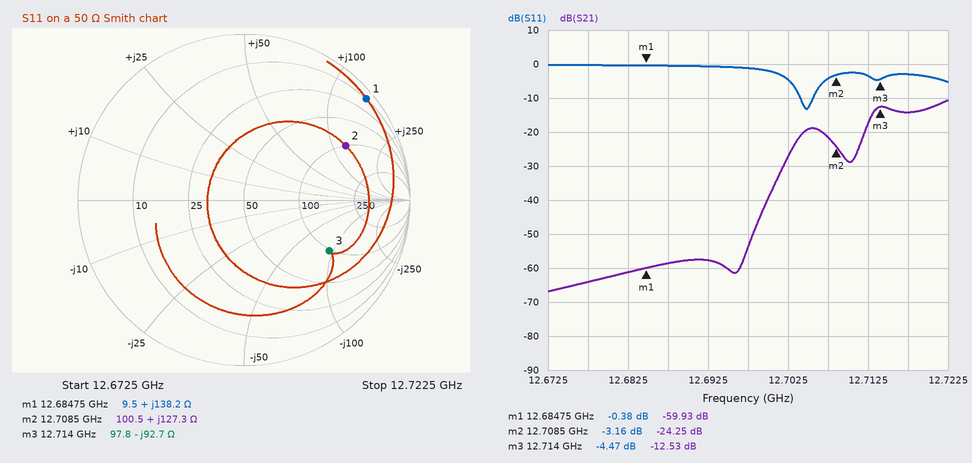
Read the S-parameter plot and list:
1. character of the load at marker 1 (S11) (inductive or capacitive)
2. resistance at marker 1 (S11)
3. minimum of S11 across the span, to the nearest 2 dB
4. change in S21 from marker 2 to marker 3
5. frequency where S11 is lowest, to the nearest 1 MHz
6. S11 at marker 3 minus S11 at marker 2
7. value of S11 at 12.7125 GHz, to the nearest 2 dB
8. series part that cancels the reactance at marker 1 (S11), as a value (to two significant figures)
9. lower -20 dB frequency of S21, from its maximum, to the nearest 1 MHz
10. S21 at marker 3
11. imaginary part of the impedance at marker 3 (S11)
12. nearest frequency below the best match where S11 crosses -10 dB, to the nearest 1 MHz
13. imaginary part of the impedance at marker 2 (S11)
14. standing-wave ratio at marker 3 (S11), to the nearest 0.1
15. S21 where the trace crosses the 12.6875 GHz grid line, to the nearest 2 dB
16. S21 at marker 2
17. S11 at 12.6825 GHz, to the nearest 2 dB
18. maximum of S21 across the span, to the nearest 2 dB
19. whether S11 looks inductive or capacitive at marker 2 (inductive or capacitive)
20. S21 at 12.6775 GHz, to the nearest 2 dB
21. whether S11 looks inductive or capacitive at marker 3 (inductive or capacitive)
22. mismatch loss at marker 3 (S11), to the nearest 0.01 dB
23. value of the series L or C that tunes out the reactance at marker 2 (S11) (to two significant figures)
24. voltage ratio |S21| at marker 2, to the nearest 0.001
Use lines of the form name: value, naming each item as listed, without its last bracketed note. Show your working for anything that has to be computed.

character of the load at marker 1 (S11): inductive
resistance at marker 1: 9.5 Ω
minimum of S11 across the span, to the nearest 2 dB: -14 dB
change in S21 from marker 2 to marker 3: -12.53 − (-24.25) = 11.72 dB
frequency where S11 is lowest, to the nearest 1 MHz: 12.705 GHz
S11 at marker 3 minus S11 at marker 2: -4.47 − (-3.16) = -1.31 dB
value of S11 at 12.7125 GHz, to the nearest 2 dB: -4 dB
series part that cancels the reactance at marker 1 (S11), as a value: C = 1/(2π × 12.68475 GHz × 138.2 Ω) ≈ 91 fF
lower -20 dB frequency of S21, from its maximum, to the nearest 1 MHz: 12.702 GHz
S21 at marker 3: -12.53 dB
imaginary part of the impedance at marker 3: -92.7 Ω
nearest frequency below the best match where S11 crosses -10 dB, to the nearest 1 MHz: 12.704 GHz
imaginary part of the impedance at marker 2: +127.3 Ω
standing-wave ratio at marker 3 (S11), to the nearest 0.1: 4.0
S21 where the trace crosses the 12.6875 GHz grid line, to the nearest 2 dB: -58 dB
S21 at marker 2: -24.25 dB
S11 at 12.6825 GHz, to the nearest 2 dB: 0 dB
maximum of S21 across the span, to the nearest 2 dB: -10 dB
whether S11 looks inductive or capacitive at marker 2: inductive
S21 at 12.6775 GHz, to the nearest 2 dB: -64 dB
whether S11 looks inductive or capacitive at marker 3: capacitive
mismatch loss at marker 3 (S11), to the nearest 0.01 dB: −10 log10(1 − 10^(-4.47/10)) ≈ 1.92 dB
value of the series L or C that tunes out the reactance at marker 2 (S11): C = 1/(2π × 12.7085 GHz × 127.3 Ω) ≈ 98 fF
voltage ratio |S21| at marker 2, to the nearest 0.001: 10^(-24.25/20) ≈ 0.061
